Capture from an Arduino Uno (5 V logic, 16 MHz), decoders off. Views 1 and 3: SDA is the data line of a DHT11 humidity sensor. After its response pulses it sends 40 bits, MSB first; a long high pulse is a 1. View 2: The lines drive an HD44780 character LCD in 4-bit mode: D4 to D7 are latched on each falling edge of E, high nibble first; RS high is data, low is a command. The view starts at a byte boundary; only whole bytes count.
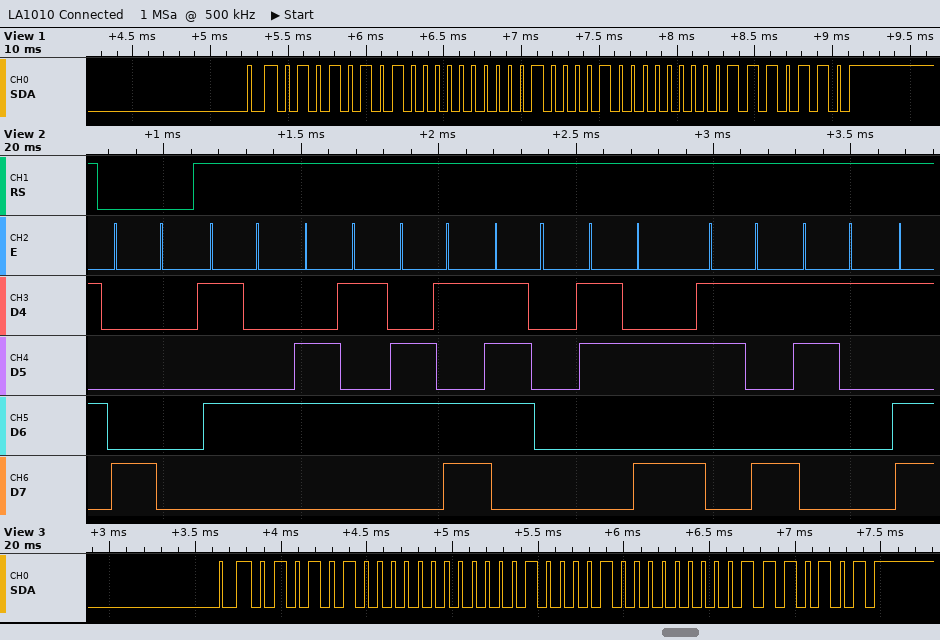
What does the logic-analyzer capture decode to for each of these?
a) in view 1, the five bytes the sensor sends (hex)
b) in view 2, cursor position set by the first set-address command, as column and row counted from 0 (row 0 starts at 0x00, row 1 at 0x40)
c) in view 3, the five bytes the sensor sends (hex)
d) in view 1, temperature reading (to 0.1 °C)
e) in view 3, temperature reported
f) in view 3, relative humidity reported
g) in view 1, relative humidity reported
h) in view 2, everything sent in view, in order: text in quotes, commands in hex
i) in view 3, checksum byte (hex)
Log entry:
55 00 21 00 76
column 0, row 0
54 00 21 00 75
33.0 °C
33.0 °C
84 %
85 %
0x80 "Temp:91"
0x75
